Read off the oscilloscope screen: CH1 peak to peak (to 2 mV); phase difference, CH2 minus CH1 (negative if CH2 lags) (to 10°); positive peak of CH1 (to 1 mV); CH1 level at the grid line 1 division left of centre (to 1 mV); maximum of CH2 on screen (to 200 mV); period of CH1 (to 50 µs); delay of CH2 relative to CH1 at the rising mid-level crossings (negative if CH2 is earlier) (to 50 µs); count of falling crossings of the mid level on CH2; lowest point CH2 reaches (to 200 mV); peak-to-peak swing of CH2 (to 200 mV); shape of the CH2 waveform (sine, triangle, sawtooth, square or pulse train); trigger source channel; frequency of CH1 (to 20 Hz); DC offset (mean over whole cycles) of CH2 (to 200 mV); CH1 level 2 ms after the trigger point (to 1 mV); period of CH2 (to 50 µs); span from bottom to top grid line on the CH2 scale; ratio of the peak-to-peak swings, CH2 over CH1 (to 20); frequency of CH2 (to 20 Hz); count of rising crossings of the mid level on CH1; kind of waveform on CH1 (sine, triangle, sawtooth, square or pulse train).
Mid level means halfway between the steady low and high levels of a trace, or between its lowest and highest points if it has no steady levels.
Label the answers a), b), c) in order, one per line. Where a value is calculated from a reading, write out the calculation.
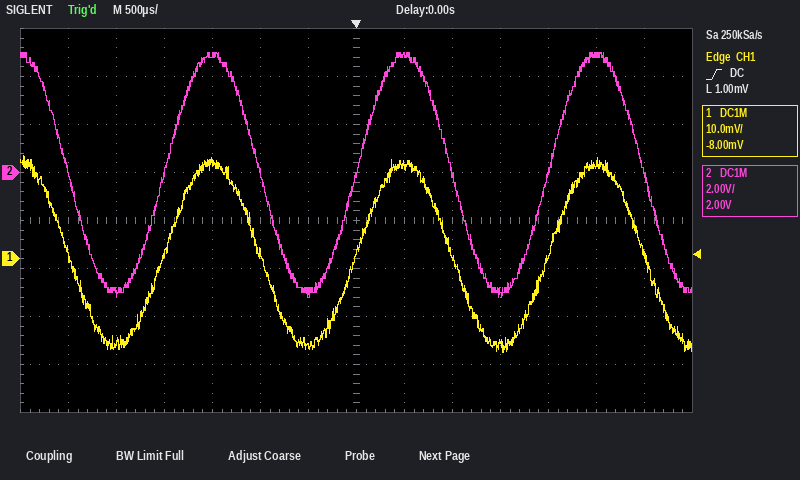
a) 42 mV
b) −360° × (0 µs) / 2.00 ms ≈ 0°
c) 22 mV
d) -18 mV
e) 5.0 V
f) 2.00 ms
g) 0 µs
h) 4
i) -5.2 V
j) 5.0 V − (-5.2 V) = 10.2 V
k) sine
l) CH1
m) 1 / 2.00 ms ≈ 500 Hz
n) (5.0 V + (-5.2 V)) / 2 ≈ 0.0 V
o) 0 mV
p) 2.00 ms
q) 16 V
r) 10.2 V / 42 mV ≈ 243, so 240 to the nearest 20
s) 1 / 2.00 ms ≈ 500 Hz
t) 3
u) sine
